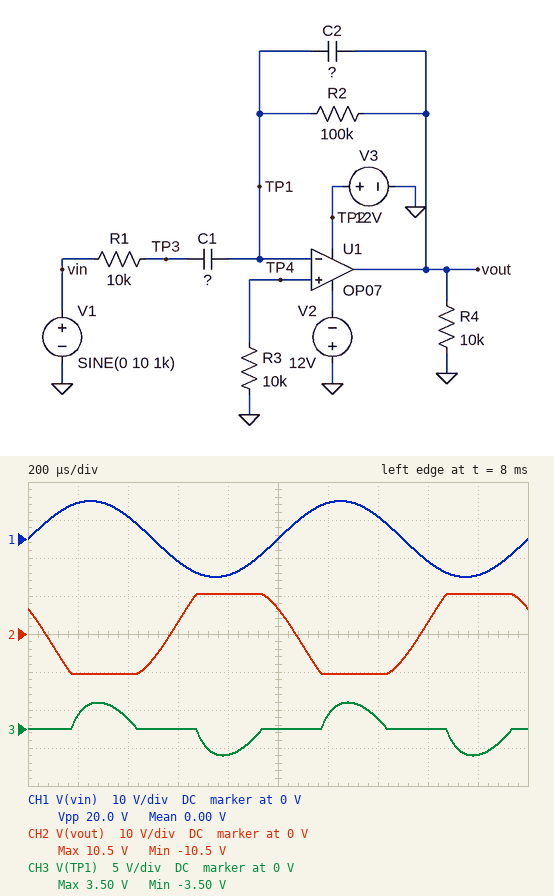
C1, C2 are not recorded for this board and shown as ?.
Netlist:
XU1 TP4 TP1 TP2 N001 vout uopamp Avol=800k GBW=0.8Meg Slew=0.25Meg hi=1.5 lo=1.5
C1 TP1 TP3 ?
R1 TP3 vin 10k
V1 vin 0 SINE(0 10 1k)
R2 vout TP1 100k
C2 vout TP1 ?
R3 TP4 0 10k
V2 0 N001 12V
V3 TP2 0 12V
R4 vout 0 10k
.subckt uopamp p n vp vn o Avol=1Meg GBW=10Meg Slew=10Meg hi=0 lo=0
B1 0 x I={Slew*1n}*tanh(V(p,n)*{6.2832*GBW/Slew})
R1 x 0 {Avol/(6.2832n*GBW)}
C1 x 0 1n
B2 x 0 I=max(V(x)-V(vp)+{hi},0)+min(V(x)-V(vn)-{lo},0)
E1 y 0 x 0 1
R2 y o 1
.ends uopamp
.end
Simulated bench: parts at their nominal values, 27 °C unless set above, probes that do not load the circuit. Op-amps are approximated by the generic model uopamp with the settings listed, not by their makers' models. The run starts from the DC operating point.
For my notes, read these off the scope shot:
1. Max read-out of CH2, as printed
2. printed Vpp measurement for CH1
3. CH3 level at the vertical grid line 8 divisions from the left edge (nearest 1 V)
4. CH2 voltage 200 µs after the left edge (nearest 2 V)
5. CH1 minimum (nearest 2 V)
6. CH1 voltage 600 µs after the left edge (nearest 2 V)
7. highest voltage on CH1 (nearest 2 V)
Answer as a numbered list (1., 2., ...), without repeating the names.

1. 10.5 V
2. 20.0 V
3. 0 V
4. -10 V
5. -10 V
6. -6 V
7. 10 V
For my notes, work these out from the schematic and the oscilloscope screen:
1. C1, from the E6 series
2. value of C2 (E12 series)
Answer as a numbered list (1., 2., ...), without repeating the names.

1. 15 nF
2. 5.6 nF
